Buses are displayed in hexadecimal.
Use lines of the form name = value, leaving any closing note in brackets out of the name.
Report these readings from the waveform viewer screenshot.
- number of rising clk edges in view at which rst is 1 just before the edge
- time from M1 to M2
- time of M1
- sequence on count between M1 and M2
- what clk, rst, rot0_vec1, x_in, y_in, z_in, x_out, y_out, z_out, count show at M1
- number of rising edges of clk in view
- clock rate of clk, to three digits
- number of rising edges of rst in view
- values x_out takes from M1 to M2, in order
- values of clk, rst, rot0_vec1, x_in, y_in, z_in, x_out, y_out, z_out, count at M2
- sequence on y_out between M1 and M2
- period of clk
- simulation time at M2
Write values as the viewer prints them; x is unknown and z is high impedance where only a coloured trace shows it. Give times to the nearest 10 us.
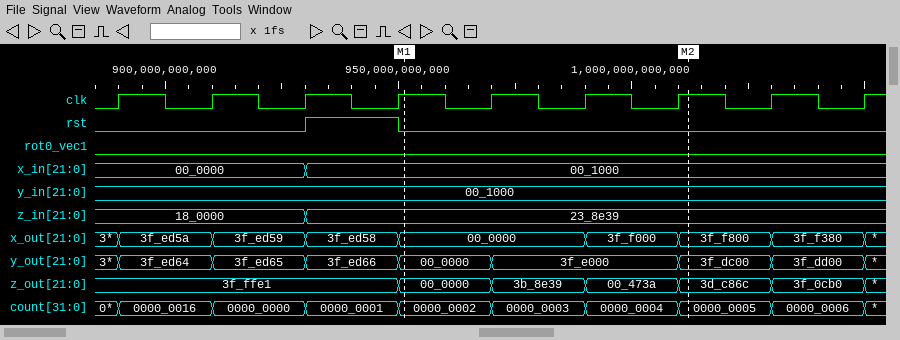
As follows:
number of rising clk edges in view at which rst is 1 just before the edge = 1
time from M1 to M2 = 60 us
time of M1 = 950 us
sequence on count between M1 and M2 = 0000_0002, 0000_0003, 0000_0004, 0000_0005
what clk, rst, rot0_vec1, x_in, y_in, z_in, x_out, y_out, z_out, count show at M1 = clk=1, rst=0, rot0_vec1=0, x_in=00_1000, y_in=00_1000, z_in=23_8e39, x_out=00_0000, y_out=00_0000, z_out=00_0000, count=0000_0002
number of rising edges of clk in view = 9
clock rate of clk, to three digits = 50.0 kHz
number of rising edges of rst in view = 1
values x_out takes from M1 to M2, in order = 00_0000, 3f_f000, 3f_f800
values of clk, rst, rot0_vec1, x_in, y_in, z_in, x_out, y_out, z_out, count at M2 = clk=1, rst=0, rot0_vec1=0, x_in=00_1000, y_in=00_1000, z_in=23_8e39, x_out=3f_f800, y_out=3f_dc00, z_out=3d_c86c, count=0000_0005
sequence on y_out between M1 and M2 = 00_0000, 3f_e000, 3f_dc00
period of clk = 20 us
simulation time at M2 = 1010 us
